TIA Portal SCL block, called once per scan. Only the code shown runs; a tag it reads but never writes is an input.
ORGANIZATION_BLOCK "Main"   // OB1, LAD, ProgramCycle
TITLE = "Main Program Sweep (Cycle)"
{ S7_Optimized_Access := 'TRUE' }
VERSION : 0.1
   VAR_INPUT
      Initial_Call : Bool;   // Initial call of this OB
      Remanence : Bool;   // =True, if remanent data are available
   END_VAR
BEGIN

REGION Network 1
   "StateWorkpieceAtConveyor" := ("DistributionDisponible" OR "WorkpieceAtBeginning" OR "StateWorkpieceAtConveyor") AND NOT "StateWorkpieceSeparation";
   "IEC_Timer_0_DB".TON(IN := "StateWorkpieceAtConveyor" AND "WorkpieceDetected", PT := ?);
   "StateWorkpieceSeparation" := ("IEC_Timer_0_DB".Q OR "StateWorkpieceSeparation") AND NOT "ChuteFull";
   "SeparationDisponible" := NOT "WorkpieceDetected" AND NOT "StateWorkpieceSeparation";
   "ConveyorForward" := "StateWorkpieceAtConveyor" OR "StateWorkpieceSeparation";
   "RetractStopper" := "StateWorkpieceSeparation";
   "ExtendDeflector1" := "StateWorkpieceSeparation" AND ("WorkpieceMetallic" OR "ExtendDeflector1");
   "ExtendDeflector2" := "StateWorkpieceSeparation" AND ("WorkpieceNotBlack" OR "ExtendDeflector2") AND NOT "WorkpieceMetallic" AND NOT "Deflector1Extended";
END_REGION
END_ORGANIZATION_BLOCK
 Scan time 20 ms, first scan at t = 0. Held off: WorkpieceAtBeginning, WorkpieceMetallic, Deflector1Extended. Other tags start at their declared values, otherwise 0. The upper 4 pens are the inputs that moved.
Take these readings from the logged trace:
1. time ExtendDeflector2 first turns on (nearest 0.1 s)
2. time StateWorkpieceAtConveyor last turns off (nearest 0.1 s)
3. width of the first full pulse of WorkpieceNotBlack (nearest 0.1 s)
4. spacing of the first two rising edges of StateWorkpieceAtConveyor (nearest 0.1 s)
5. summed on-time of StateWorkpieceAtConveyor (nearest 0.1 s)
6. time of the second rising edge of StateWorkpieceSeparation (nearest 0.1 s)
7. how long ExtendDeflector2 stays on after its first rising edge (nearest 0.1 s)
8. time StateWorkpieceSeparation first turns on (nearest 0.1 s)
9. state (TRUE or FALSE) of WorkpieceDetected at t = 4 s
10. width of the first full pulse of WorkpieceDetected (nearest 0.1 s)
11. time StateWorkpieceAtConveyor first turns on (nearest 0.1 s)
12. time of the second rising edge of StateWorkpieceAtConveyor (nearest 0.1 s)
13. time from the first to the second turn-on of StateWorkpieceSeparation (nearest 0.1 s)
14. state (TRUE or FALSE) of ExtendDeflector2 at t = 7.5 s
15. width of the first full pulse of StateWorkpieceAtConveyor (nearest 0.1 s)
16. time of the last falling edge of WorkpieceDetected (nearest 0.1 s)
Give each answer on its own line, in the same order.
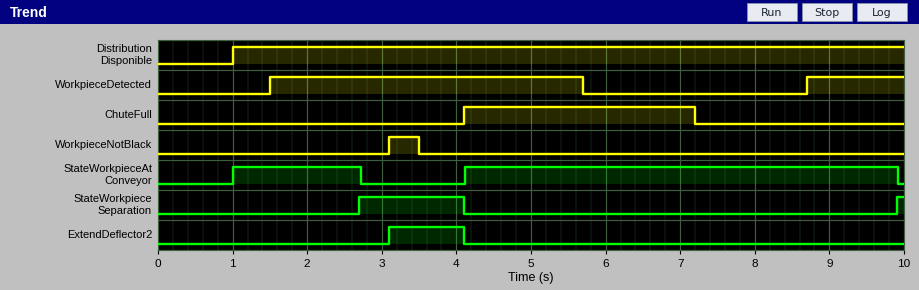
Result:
3.1 s
9.9 s
0.4 s
3.1 s
7.5 s
9.9 s
1.0 s
2.7 s
TRUE
4.2 s
1.0 s
4.1 s
7.2 s
FALSE
1.7 s
5.7 s
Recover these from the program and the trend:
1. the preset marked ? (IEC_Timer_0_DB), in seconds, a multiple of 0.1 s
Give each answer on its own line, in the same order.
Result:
1.2 s
